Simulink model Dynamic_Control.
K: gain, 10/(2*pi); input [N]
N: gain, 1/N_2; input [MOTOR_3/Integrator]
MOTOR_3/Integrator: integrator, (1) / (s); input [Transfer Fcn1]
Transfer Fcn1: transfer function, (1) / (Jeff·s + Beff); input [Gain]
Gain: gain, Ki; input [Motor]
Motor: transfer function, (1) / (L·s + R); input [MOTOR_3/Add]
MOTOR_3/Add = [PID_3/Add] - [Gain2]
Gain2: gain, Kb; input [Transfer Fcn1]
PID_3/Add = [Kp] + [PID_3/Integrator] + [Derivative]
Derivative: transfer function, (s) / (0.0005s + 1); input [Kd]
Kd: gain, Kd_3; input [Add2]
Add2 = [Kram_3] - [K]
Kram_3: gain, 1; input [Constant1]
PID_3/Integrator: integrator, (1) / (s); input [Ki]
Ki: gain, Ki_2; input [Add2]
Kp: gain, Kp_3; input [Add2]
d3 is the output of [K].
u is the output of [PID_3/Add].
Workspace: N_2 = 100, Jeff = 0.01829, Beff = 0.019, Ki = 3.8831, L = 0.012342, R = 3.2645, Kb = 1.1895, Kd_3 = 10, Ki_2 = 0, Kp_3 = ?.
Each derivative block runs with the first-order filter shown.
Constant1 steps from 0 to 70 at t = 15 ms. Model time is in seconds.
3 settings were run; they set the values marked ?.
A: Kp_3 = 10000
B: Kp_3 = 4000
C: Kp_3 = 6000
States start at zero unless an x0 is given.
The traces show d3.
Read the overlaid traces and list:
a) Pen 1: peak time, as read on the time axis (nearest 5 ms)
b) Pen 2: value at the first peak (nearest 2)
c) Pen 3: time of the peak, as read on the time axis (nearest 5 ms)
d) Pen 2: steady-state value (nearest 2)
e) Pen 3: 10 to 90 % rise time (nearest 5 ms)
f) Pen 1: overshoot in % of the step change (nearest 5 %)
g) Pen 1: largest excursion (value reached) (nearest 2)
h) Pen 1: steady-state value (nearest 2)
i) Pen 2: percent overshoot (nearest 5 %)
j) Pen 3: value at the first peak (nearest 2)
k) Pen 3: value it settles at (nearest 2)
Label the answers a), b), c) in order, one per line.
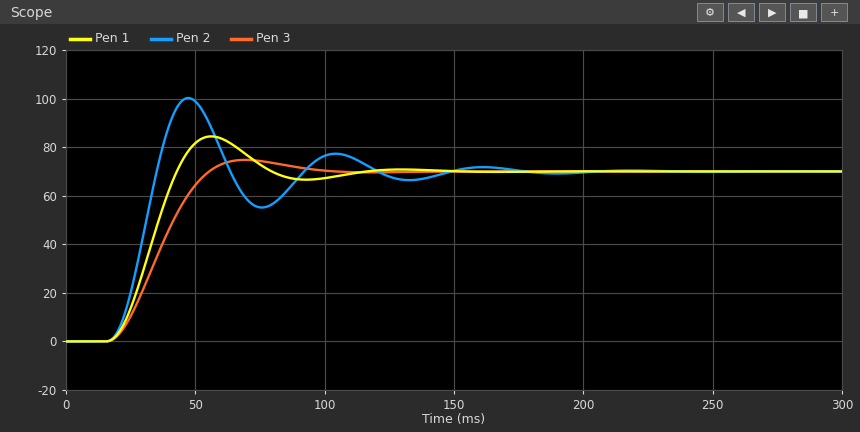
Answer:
a) 55 ms
b) 100
c) 70 ms
d) 70
e) 25 ms
f) 20 %
g) 84
h) 70
i) 45 %
j) 74
k) 70
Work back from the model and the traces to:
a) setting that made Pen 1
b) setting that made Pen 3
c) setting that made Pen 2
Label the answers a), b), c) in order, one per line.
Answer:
a) C
b) B
c) A
